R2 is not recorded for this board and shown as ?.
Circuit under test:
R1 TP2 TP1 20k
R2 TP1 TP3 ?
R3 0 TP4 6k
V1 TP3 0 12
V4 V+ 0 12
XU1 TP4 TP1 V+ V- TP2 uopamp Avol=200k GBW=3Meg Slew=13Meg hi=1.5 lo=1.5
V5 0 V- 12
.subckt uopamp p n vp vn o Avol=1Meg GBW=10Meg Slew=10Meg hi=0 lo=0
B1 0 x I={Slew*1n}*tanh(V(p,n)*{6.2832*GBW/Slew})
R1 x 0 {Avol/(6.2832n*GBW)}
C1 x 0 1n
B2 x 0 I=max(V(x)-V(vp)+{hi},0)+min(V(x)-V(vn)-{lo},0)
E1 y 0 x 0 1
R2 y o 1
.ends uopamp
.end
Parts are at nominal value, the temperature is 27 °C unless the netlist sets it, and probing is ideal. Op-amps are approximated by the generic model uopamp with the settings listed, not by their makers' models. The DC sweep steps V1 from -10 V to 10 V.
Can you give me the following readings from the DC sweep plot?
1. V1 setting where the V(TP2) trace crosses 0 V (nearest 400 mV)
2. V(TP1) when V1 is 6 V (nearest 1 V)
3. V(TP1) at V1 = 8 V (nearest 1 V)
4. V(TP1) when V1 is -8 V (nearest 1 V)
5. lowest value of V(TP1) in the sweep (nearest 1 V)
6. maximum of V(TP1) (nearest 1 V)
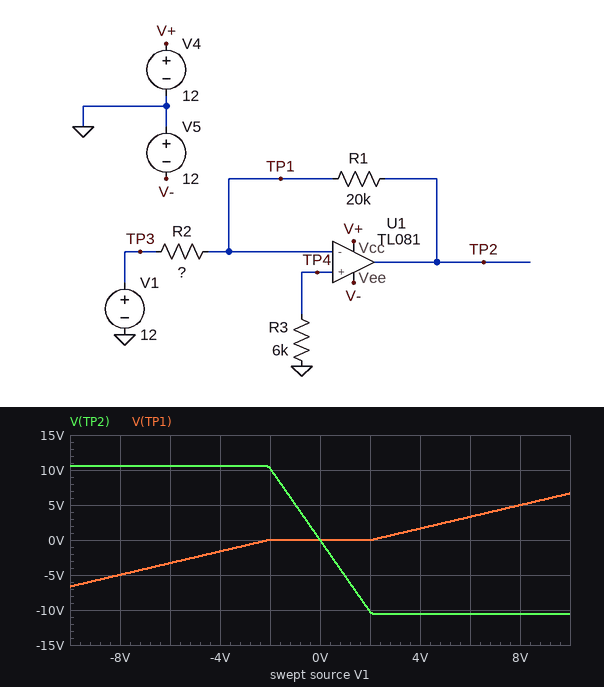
0 V
3 V
5 V
-5 V
-7 V
7 V
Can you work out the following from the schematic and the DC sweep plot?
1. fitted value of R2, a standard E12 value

3.9 kΩ
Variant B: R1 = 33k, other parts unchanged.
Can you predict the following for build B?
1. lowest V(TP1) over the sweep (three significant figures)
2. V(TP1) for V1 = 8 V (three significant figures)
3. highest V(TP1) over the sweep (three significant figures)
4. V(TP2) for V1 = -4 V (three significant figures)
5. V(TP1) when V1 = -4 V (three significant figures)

-7.83 V
6.04 V
7.83 V
10.5 V
-2.47 V
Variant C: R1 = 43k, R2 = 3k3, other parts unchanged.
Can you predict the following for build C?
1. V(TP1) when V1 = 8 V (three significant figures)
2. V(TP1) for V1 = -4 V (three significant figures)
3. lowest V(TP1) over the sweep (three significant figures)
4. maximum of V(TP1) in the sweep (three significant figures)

6.68 V
-2.97 V
-8.54 V
8.54 V
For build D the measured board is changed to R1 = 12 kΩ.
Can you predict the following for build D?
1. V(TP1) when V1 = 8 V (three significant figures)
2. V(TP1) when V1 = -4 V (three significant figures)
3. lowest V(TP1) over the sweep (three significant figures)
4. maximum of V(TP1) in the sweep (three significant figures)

3.46 V
-442 mV
-4.97 V
4.97 V
